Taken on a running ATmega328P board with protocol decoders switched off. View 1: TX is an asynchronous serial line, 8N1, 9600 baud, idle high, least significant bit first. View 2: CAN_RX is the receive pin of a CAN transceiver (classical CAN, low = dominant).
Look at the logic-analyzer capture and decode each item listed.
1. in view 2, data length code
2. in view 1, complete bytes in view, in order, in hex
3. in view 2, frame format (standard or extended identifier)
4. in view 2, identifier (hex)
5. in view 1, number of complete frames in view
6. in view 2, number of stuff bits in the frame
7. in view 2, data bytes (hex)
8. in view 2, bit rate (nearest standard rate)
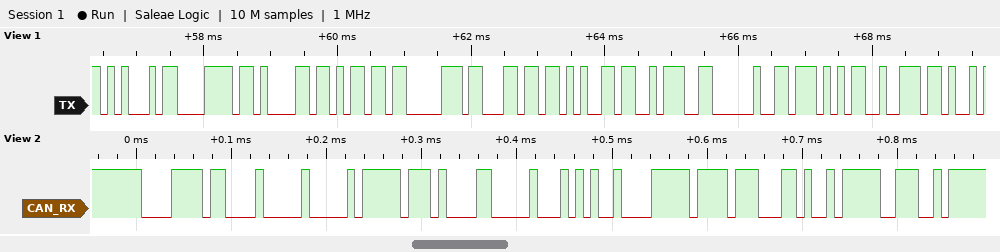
8
45 78 61 6D 70 6C 65 3A 20 57 72
standard
0x0F6
11
6
00 FF 43 00 A9 0F FB 8D
125 kbit/s
